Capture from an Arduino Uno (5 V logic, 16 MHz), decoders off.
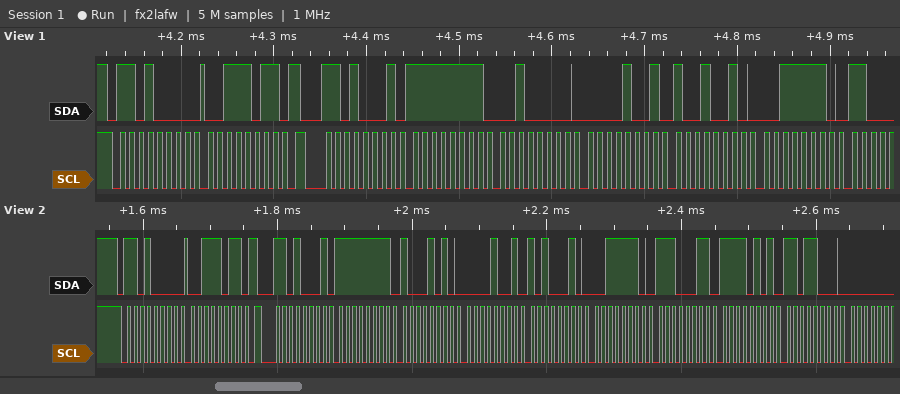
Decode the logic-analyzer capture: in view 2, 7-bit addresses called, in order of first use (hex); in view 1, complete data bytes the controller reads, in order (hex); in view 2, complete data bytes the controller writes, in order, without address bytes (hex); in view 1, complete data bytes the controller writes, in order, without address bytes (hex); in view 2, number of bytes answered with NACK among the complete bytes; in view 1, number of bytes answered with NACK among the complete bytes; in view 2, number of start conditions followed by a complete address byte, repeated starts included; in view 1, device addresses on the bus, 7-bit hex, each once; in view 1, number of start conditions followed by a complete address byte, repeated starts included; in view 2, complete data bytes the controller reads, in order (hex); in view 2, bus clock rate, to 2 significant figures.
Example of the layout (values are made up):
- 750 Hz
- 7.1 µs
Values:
- 0x68
- FF 20 09 92 3E
- 3B
- 3B
- 0
- 0
- 2
- 0x68
- 2
- FF 8A 09 A2 3E E3 F5 D8
- 100 kHz
